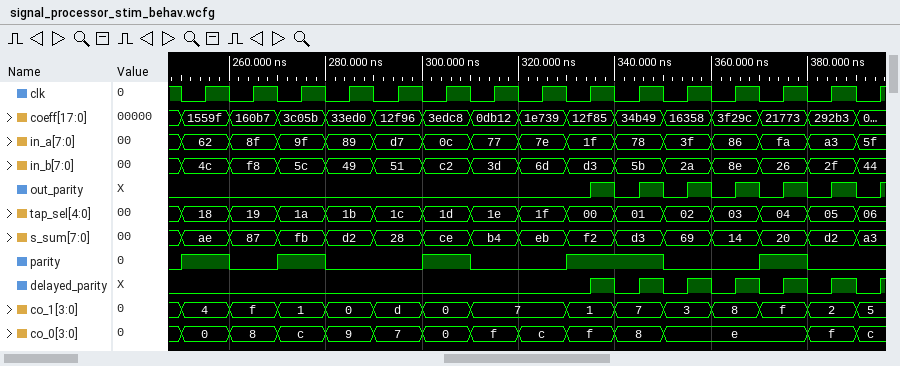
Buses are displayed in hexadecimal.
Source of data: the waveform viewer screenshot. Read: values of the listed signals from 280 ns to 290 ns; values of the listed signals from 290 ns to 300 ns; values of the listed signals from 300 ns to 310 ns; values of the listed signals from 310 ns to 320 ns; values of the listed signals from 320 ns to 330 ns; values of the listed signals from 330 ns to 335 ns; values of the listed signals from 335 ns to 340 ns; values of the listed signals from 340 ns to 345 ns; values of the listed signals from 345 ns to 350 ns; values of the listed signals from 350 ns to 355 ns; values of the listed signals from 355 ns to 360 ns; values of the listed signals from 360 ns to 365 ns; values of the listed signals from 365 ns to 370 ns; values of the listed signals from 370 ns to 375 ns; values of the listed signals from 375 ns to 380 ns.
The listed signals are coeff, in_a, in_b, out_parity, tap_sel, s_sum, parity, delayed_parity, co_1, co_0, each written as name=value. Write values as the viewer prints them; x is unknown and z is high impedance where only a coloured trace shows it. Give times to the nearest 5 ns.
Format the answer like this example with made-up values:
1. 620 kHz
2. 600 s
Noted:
1. coeff=33ed0, in_a=89, in_b=49, out_parity=0, tap_sel=1b, s_sum=d2, parity=0, delayed_parity=0, co_1=0, co_0=9
2. coeff=12f96, in_a=d7, in_b=51, out_parity=0, tap_sel=1c, s_sum=28, parity=0, delayed_parity=0, co_1=d, co_0=7
3. coeff=3edc8, in_a=0c, in_b=c2, out_parity=0, tap_sel=1d, s_sum=ce, parity=1, delayed_parity=0, co_1=0, co_0=0
4. coeff=0db12, in_a=77, in_b=3d, out_parity=0, tap_sel=1e, s_sum=b4, parity=0, delayed_parity=0, co_1=7, co_0=f
5. coeff=1e739, in_a=7e, in_b=6d, out_parity=0, tap_sel=1f, s_sum=eb, parity=0, delayed_parity=0, co_1=7, co_0=c
6. coeff=12f85, in_a=1f, in_b=d3, out_parity=0, tap_sel=00, s_sum=f2, parity=1, delayed_parity=0, co_1=1, co_0=f
7. coeff=12f85, in_a=1f, in_b=d3, out_parity=1, tap_sel=00, s_sum=f2, parity=1, delayed_parity=1, co_1=1, co_0=f
8. coeff=34b49, in_a=78, in_b=5b, out_parity=0, tap_sel=01, s_sum=d3, parity=1, delayed_parity=0, co_1=7, co_0=8
9. coeff=34b49, in_a=78, in_b=5b, out_parity=1, tap_sel=01, s_sum=d3, parity=1, delayed_parity=1, co_1=7, co_0=8
10. coeff=16358, in_a=3f, in_b=2a, out_parity=0, tap_sel=02, s_sum=69, parity=0, delayed_parity=0, co_1=3, co_0=e
11. coeff=16358, in_a=3f, in_b=2a, out_parity=1, tap_sel=02, s_sum=69, parity=0, delayed_parity=1, co_1=3, co_0=e
12. coeff=3f29c, in_a=86, in_b=8e, out_parity=0, tap_sel=03, s_sum=14, parity=0, delayed_parity=0, co_1=8, co_0=e
13. coeff=3f29c, in_a=86, in_b=8e, out_parity=1, tap_sel=03, s_sum=14, parity=0, delayed_parity=1, co_1=8, co_0=e
14. coeff=21773, in_a=fa, in_b=26, out_parity=0, tap_sel=04, s_sum=20, parity=1, delayed_parity=0, co_1=f, co_0=e
15. coeff=21773, in_a=fa, in_b=26, out_parity=1, tap_sel=04, s_sum=20, parity=1, delayed_parity=1, co_1=f, co_0=e
